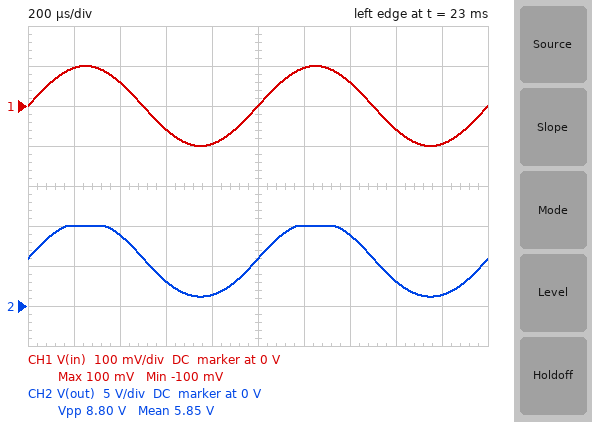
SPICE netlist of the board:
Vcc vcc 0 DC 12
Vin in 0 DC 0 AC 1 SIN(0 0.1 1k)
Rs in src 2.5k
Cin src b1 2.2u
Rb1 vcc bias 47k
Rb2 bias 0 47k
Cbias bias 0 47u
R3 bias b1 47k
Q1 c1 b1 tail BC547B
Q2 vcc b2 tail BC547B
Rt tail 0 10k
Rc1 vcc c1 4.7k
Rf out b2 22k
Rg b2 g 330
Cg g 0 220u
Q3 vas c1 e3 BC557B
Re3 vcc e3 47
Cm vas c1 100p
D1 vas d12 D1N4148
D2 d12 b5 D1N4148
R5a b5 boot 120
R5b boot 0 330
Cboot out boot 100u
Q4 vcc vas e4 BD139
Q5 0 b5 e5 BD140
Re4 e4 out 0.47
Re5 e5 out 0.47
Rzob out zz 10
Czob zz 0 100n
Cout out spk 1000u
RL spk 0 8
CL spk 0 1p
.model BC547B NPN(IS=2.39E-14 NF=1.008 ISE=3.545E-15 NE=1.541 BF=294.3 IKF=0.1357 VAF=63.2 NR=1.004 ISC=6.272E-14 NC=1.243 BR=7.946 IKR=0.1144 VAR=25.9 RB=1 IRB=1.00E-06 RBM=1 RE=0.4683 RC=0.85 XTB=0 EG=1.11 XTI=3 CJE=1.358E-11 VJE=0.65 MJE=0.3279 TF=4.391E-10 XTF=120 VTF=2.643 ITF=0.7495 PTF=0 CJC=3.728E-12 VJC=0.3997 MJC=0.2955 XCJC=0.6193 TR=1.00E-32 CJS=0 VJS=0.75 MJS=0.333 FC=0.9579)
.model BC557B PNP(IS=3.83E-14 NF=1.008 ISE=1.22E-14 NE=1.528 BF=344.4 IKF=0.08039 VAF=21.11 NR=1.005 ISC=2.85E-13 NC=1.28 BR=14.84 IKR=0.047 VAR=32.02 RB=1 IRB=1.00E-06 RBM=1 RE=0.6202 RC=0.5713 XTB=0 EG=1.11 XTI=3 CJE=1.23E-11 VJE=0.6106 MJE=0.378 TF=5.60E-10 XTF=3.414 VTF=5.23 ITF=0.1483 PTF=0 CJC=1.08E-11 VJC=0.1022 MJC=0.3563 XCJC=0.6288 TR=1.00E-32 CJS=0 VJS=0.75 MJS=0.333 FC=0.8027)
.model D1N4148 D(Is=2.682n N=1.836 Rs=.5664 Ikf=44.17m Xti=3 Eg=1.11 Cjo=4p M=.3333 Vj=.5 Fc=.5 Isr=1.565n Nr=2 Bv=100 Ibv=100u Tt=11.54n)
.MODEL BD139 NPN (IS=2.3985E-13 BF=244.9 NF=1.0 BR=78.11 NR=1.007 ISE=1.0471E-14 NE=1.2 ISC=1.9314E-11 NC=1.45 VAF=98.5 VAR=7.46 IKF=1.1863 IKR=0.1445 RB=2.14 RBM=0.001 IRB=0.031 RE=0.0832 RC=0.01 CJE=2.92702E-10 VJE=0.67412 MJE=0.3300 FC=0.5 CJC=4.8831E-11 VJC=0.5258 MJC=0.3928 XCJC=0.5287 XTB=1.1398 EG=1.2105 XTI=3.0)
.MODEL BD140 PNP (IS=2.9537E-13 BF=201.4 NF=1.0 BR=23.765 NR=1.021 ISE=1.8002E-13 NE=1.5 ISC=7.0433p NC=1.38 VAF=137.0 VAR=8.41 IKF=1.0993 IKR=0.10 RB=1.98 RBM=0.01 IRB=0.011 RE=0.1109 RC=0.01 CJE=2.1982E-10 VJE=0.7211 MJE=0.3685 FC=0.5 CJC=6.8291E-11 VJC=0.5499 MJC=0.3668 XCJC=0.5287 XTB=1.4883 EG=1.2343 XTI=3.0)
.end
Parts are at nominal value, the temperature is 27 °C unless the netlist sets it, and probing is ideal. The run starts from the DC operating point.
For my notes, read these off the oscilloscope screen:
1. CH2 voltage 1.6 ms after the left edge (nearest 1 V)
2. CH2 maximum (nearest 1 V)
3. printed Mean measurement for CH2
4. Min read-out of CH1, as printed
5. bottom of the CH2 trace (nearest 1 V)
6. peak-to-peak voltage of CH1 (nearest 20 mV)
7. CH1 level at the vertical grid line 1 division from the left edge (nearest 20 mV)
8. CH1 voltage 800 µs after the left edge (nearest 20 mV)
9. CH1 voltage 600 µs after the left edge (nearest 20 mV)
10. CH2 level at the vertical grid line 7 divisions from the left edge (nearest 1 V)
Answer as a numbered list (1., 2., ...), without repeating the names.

1. 3 V
2. 10 V
3. 5.85 V
4. -100 mV
5. 1 V
6. 200 mV
7. 100 mV
8. -100 mV
9. -60 mV
10. 9 V
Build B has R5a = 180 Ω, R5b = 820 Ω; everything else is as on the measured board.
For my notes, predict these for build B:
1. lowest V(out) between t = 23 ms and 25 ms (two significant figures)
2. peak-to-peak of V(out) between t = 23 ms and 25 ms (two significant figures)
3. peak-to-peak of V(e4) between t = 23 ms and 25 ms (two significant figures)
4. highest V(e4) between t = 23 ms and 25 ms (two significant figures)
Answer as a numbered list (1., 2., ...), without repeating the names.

1. 2.4 V
2. 8.0 V
3. 8.2 V
4. 11 V
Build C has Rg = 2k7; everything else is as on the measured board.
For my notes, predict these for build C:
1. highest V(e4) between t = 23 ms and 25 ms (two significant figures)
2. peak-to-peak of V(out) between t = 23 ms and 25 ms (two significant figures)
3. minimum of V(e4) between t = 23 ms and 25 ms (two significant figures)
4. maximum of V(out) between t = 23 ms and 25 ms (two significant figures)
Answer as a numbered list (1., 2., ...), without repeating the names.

1. 6.9 V
2. 1.7 V
3. 5.1 V
4. 6.8 V
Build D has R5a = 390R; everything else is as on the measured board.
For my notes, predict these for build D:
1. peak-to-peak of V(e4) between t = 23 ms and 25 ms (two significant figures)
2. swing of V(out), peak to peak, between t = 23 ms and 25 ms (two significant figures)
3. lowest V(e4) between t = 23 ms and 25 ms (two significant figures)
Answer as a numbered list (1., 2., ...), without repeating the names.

1. 9.5 V
2. 9.2 V
3. 1.0 V
